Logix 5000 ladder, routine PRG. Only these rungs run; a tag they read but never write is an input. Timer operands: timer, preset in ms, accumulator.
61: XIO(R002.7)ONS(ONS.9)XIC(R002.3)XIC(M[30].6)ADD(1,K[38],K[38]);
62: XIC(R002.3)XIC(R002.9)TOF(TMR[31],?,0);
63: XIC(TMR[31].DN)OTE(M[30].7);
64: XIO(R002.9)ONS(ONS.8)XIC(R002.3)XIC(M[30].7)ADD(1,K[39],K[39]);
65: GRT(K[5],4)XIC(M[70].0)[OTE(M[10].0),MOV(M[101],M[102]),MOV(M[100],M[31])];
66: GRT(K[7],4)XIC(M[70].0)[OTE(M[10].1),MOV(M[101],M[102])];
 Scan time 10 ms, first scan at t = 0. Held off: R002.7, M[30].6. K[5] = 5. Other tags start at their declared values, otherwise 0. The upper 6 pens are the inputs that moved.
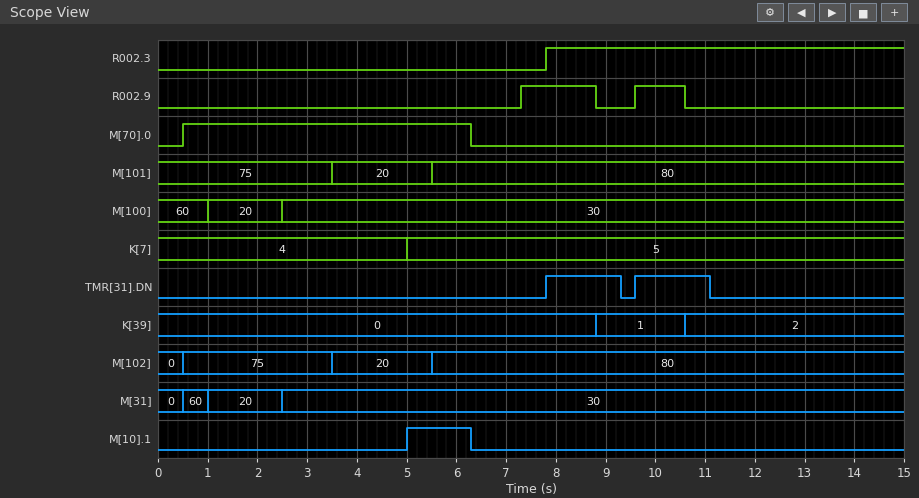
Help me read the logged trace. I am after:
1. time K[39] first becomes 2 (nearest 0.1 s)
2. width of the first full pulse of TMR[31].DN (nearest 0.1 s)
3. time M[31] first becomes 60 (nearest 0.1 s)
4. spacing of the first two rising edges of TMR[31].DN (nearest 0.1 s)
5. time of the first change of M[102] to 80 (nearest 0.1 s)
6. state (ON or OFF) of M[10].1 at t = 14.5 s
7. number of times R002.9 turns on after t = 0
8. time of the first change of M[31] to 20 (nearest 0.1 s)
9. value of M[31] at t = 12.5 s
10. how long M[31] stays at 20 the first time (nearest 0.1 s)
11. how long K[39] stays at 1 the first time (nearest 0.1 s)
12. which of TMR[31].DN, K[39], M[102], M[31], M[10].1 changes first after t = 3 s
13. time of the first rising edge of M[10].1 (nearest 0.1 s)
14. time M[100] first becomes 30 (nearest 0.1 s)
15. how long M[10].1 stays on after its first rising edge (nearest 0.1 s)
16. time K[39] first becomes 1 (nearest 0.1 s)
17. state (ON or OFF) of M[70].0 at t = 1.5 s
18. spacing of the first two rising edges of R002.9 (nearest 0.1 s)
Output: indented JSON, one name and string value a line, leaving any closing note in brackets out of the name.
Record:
{
  "time K[39] first becomes 2": "10.6 s",
  "width of the first full pulse of TMR[31].DN": "1.5 s",
  "time M[31] first becomes 60": "0.5 s",
  "spacing of the first two rising edges of TMR[31].DN": "1.8 s",
  "time of the first change of M[102] to 80": "5.5 s",
  "state (ON or OFF) of M[10].1 at t = 14.5 s": "OFF",
  "number of times R002.9 turns on after t = 0": "2",
  "time of the first change of M[31] to 20": "1.0 s",
  "value of M[31] at t = 12.5 s": "30",
  "how long M[31] stays at 20 the first time": "1.5 s",
  "how long K[39] stays at 1 the first time": "1.8 s",
  "which of TMR[31].DN, K[39], M[102], M[31], M[10].1 changes first after t = 3 s": "M[102]",
  "time of the first rising edge of M[10].1": "5.0 s",
  "time M[100] first becomes 30": "2.5 s",
  "how long M[10].1 stays on after its first rising edge": "1.3 s",
  "time K[39] first becomes 1": "8.8 s",
  "state (ON or OFF) of M[70].0 at t = 1.5 s": "ON",
  "spacing of the first two rising edges of R002.9": "2.3 s"
}
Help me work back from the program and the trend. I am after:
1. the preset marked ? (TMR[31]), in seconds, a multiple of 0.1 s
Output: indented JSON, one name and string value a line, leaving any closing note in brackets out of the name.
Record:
{
  "the preset marked ? (TMR[31]), in seconds, a multiple of 0.1 s": "0.5 s"
}
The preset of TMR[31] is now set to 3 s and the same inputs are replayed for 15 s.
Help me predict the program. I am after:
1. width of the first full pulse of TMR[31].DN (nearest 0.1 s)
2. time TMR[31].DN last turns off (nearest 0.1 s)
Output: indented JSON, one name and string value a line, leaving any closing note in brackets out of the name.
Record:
{
  "width of the first full pulse of TMR[31].DN": "5.8 s",
  "time TMR[31].DN last turns off": "13.6 s"
}
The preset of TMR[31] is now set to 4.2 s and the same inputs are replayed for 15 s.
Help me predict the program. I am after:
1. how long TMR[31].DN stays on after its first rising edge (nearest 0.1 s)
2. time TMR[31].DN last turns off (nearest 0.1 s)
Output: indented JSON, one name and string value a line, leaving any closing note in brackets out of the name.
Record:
{
  "how long TMR[31].DN stays on after its first rising edge": "7.0 s",
  "time TMR[31].DN last turns off": "14.8 s"
}
